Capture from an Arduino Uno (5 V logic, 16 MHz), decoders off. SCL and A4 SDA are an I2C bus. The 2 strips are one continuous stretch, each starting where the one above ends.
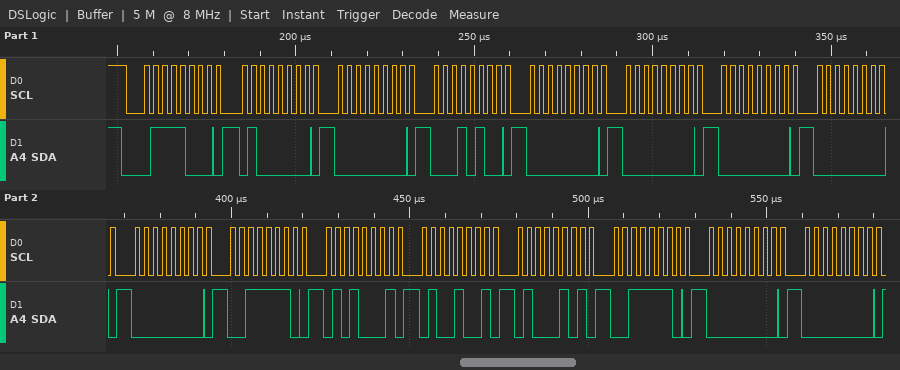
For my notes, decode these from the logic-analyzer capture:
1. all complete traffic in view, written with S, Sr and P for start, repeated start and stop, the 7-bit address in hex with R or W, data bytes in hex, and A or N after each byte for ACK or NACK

S 3CW A 40 A 00 A 14 A 00 A 00 A 00 A 00 A 00 A 3E A 51 A 49 A 45 A 3E A 00 A 00 A
